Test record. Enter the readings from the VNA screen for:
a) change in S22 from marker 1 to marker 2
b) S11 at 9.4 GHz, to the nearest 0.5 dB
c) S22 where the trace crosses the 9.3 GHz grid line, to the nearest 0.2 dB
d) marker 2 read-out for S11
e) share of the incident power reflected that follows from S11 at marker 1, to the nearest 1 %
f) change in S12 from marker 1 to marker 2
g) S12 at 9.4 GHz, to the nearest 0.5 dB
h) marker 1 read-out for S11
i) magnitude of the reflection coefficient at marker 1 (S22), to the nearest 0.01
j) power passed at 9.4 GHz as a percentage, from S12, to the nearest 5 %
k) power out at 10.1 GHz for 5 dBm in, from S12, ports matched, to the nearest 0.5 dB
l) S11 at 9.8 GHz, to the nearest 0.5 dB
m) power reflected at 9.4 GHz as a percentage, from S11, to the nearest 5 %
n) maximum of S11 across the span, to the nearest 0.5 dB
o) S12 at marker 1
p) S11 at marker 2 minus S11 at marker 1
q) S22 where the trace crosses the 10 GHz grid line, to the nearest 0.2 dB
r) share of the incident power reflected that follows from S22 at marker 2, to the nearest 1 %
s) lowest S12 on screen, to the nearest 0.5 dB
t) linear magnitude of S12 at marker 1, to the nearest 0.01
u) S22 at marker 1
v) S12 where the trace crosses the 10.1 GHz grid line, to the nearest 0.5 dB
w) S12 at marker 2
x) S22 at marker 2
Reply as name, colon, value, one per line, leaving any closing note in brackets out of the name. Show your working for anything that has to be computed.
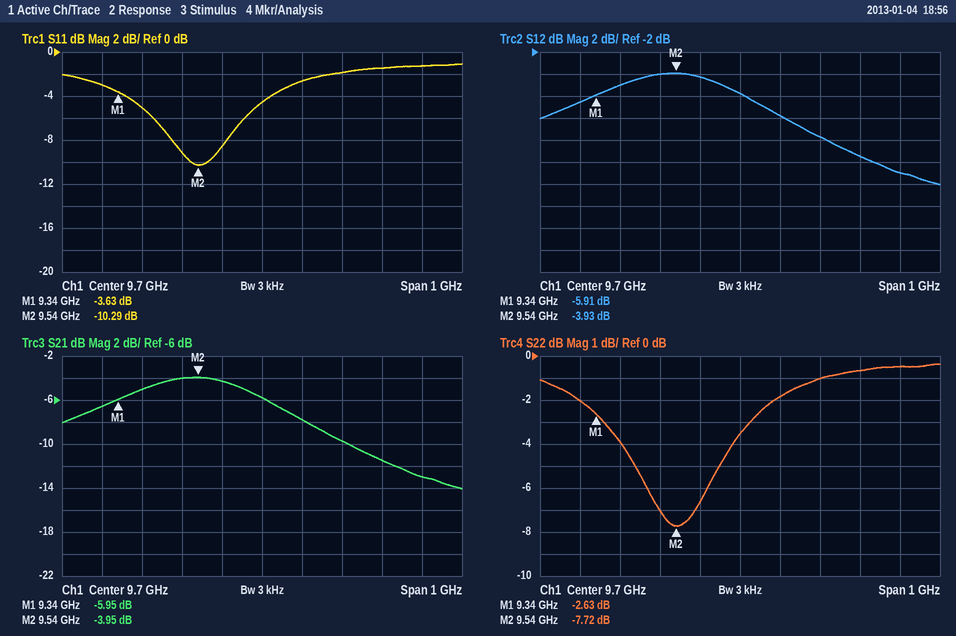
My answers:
change in S22 from marker 1 to marker 2: -7.72 − (-2.63) = -5.09 dB
S11 at 9.4 GHz, to the nearest 0.5 dB: -5.0 dB
S22 where the trace crosses the 9.3 GHz grid line, to the nearest 0.2 dB: -2.0 dB
marker 2 read-out for S11: -10.29 dB
share of the incident power reflected that follows from S11 at marker 1, to the nearest 1 %: 10^(-3.63/10) ≈ 43 %
change in S12 from marker 1 to marker 2: -3.93 − (-5.91) = 1.98 dB
S12 at 9.4 GHz, to the nearest 0.5 dB: -5.0 dB
marker 1 read-out for S11: -3.63 dB
magnitude of the reflection coefficient at marker 1 (S22), to the nearest 0.01: 10^(-2.63/20) ≈ 0.74
power passed at 9.4 GHz as a percentage, from S12, to the nearest 5 %: 10^(-5/10) ≈ 31.6 %, so 30 % to the nearest 5 %
power out at 10.1 GHz for 5 dBm in, from S12, ports matched, to the nearest 0.5 dB: 5 dBm + (-13.0 dB) = -8.0 dBm
S11 at 9.8 GHz, to the nearest 0.5 dB: -2.5 dB
power reflected at 9.4 GHz as a percentage, from S11, to the nearest 5 %: 10^(-5/10) ≈ 31.6 %, so 30 % to the nearest 5 %
maximum of S11 across the span, to the nearest 0.5 dB: -1.0 dB
S12 at marker 1: -5.91 dB
S11 at marker 2 minus S11 at marker 1: -10.29 − (-3.63) = -6.66 dB
S22 where the trace crosses the 10 GHz grid line, to the nearest 0.2 dB: -0.6 dB
share of the incident power reflected that follows from S22 at marker 2, to the nearest 1 %: 10^(-7.72/10) ≈ 17 %
lowest S12 on screen, to the nearest 0.5 dB: -14.0 dB
linear magnitude of S12 at marker 1, to the nearest 0.01: 10^(-5.91/20) ≈ 0.51
S22 at marker 1: -2.63 dB
S12 where the trace crosses the 10.1 GHz grid line, to the nearest 0.5 dB: -13.0 dB
S12 at marker 2: -3.93 dB
S22 at marker 2: -7.72 dB
